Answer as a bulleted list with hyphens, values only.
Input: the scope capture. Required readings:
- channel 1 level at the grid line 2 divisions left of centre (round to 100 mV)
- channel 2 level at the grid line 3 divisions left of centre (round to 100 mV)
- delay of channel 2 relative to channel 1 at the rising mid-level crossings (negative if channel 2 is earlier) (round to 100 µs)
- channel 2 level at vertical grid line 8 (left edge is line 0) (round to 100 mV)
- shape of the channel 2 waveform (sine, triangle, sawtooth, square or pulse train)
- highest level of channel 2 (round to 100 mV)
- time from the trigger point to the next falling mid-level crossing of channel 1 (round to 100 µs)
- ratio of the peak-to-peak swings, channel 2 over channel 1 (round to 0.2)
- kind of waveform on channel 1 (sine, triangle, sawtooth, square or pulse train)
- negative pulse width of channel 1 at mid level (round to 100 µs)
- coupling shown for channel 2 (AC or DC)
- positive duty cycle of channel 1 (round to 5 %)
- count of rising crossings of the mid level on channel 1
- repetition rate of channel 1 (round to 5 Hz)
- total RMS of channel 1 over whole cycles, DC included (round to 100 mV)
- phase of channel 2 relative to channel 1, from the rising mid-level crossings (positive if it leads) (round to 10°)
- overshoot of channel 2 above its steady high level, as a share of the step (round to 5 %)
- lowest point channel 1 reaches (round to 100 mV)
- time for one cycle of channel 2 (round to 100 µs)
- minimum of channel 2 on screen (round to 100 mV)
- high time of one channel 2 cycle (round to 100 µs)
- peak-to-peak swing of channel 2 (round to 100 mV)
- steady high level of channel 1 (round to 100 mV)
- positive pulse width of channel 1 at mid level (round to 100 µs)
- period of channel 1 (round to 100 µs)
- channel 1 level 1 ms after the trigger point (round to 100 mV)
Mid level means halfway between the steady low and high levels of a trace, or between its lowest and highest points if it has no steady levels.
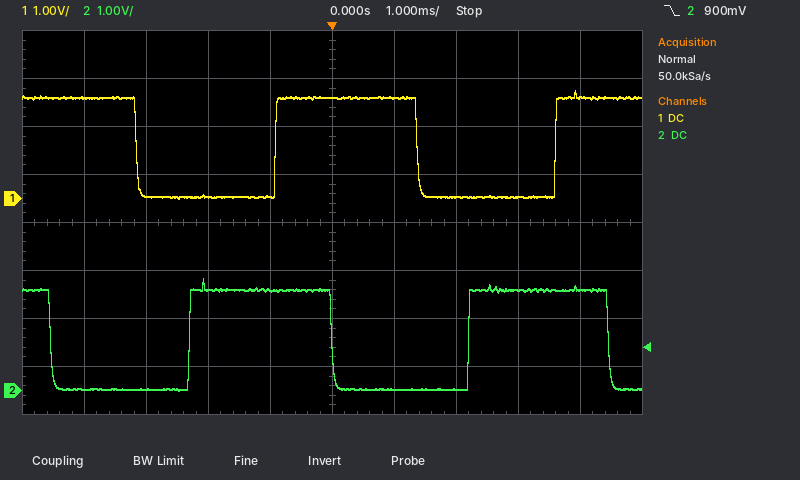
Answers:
- 0.0 V
- 0.0 V
- -1.4 ms
- 2.1 V
- square
- 2.3 V
- 1.4 ms
- 1.0
- square
- 2.2 ms
- DC
- 50 %
- 2
- 220 Hz
- 1.5 V
- +110°
- 10 %
- 0.0 V
- 4.5 ms
- 0.0 V
- 2.3 ms
- 2.3 V
- 2.1 V
- 2.3 ms
- 4.5 ms
- 2.1 V
